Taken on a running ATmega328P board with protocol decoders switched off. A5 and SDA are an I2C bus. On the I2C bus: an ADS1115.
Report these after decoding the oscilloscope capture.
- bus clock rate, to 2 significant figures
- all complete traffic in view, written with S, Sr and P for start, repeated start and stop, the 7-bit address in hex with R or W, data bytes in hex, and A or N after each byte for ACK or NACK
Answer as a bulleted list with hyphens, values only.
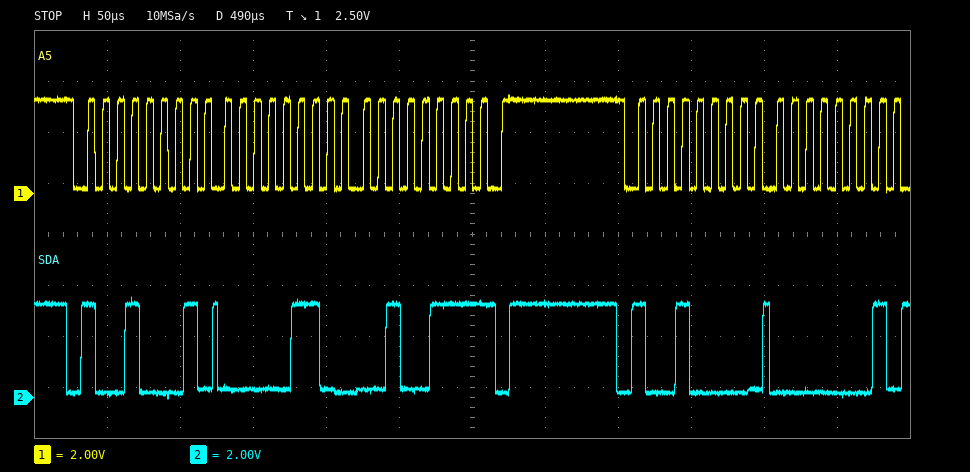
- 100 kHz
- S 48R A 06 A 27 N P S 48W A 01 A
